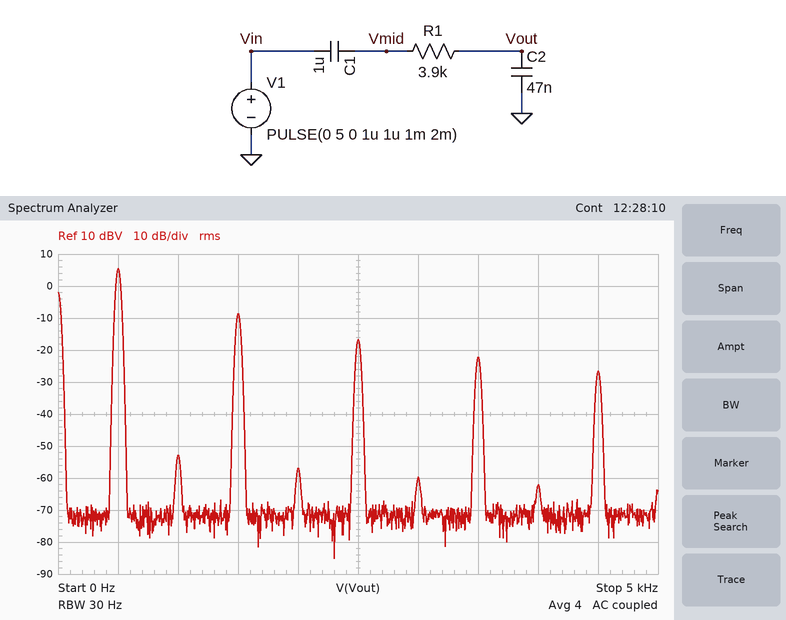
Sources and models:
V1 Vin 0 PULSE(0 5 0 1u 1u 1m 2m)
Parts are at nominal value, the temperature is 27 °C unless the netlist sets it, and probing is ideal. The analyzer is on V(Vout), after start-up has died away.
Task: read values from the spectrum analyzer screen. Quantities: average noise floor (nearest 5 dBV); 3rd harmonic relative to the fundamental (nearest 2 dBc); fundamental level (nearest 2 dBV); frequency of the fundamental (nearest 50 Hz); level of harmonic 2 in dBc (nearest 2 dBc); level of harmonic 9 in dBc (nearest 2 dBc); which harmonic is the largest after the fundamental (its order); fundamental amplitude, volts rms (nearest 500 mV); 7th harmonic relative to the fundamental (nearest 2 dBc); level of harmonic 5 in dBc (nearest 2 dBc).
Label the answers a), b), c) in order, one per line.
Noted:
a) -70 dBV
b) -14 dBc
c) 6 dBV
d) 500 Hz
e) -58 dBc
f) -32 dBc
g) 3
h) 2.0 V
i) -28 dBc
j) -22 dBc
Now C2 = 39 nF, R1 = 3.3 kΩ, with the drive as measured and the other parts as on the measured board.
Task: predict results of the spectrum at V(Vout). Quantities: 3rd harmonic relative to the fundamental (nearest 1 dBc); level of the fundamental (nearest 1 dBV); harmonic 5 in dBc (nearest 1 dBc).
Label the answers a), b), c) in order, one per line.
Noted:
a) -13 dBc
b) 6 dBV
c) -20 dBc
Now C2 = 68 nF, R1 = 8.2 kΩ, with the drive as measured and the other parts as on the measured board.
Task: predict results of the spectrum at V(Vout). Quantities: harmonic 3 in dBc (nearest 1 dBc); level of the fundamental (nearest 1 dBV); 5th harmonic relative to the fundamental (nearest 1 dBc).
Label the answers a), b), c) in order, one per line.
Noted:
a) -18 dBc
b) 1 dBV
c) -27 dBc
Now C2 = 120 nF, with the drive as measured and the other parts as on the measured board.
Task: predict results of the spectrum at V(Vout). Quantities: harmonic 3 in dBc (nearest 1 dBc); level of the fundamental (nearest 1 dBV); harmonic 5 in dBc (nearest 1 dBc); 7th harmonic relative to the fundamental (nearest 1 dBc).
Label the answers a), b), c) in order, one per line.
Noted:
a) -17 dBc
b) 2 dBV
c) -26 dBc
d) -32 dBc
